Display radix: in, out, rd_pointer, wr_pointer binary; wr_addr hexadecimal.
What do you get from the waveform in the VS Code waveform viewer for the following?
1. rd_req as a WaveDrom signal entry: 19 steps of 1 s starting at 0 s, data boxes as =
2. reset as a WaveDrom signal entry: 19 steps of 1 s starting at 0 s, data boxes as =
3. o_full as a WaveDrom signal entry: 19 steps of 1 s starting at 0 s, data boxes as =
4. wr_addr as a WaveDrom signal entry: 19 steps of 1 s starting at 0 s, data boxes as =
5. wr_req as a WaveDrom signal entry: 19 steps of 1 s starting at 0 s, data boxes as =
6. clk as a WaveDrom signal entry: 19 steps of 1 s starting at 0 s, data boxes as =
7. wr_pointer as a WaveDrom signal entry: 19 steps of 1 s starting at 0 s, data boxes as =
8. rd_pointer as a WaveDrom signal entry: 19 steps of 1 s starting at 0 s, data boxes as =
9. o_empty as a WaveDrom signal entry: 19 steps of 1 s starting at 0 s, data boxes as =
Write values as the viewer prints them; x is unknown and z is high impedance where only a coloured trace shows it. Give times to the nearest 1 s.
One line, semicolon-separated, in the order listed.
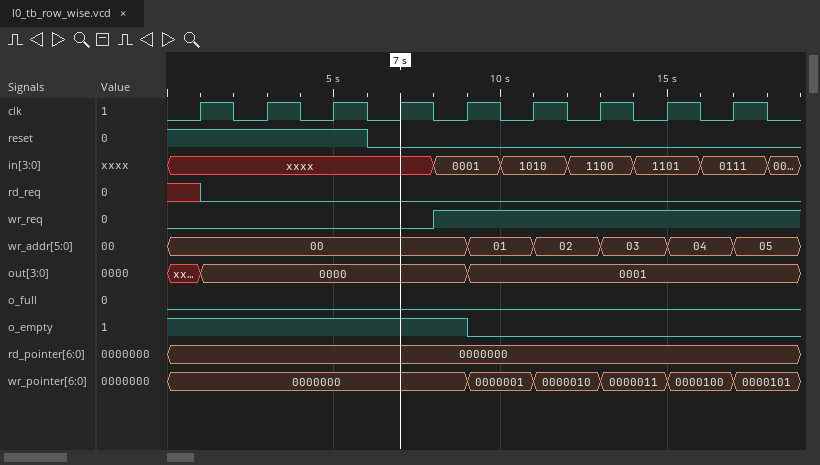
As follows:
{name: 'rd_req', wave: 'x0.................'}; {name: 'reset', wave: '1.....0............'}; {name: 'o_full', wave: '0..................'}; {name: 'wr_addr', wave: '=........=.=.=.=.=.', data: '00 01 02 03 04 05'}; {name: 'wr_req', wave: '0.......1..........'}; {name: 'clk', wave: '0101010101010101010'}; {name: 'wr_pointer', wave: '=........=.=.=.=.=.', data: '0000000 0000001 0000010 0000011 0000100 0000101'}; {name: 'rd_pointer', wave: '=..................', data: '0000000'}; {name: 'o_empty', wave: '1........0.........'}
